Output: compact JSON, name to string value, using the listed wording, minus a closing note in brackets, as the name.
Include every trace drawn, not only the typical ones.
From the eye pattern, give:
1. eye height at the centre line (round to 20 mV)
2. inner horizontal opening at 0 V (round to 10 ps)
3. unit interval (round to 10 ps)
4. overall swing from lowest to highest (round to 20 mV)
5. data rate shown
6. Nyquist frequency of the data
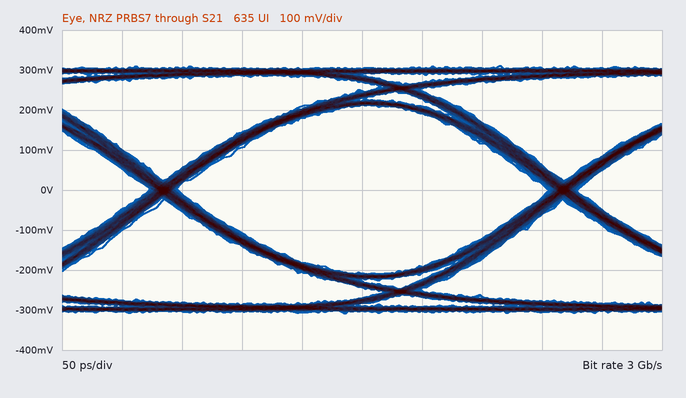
{"eye height at the centre line": "420 mV", "inner horizontal opening at 0 V": "310 ps", "unit interval": "330 ps", "overall swing from lowest to highest": "620 mV", "data rate shown": "3 Gb/s", "Nyquist frequency of the data": "1.5 GHz"}
